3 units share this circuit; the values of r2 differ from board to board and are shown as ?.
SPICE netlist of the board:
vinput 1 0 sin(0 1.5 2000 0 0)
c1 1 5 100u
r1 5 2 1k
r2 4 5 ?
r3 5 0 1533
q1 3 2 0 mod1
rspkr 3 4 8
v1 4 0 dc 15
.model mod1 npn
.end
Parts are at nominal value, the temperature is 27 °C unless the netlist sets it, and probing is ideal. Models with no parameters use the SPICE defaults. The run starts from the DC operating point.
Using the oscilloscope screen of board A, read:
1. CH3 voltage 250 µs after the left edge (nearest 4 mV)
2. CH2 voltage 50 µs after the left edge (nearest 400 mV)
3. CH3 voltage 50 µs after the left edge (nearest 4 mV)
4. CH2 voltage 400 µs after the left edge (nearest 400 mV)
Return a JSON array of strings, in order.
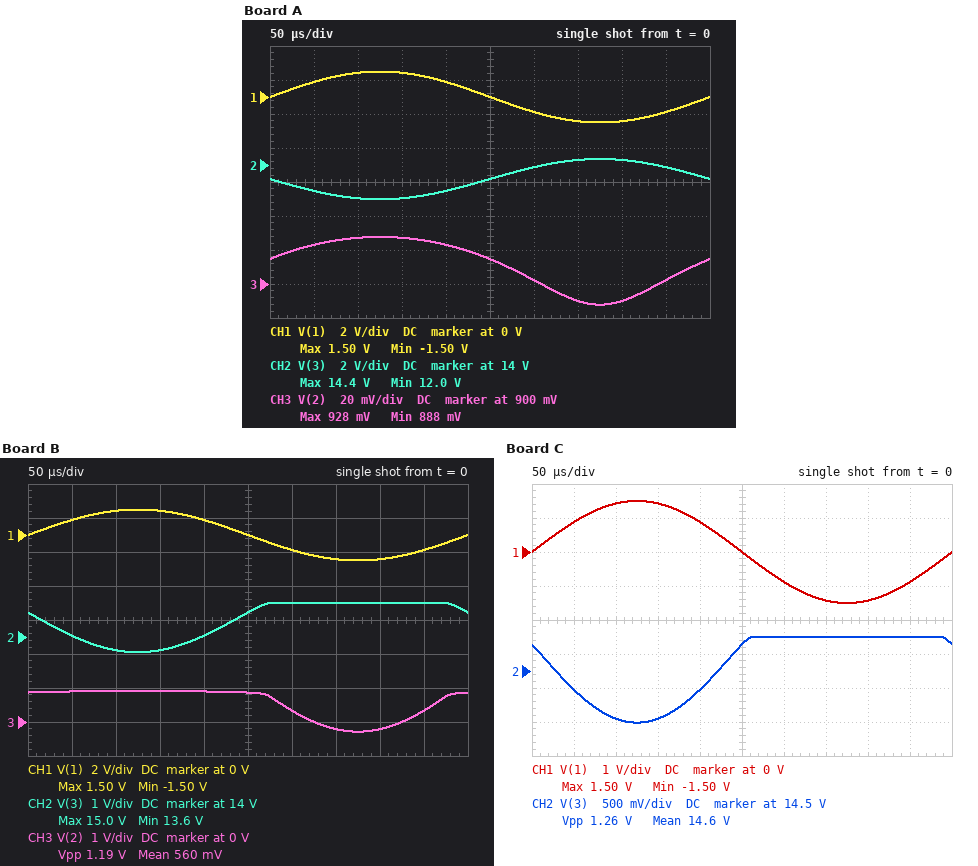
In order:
["916 mV", "12.4 V", "924 mV", "14.4 V"]
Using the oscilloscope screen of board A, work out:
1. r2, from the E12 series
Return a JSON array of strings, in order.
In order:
["2.7 kΩ"]
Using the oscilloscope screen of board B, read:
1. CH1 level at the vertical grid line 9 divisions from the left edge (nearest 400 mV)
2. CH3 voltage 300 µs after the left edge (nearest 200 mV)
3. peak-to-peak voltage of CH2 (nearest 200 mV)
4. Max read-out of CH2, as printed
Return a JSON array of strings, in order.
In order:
["-800 mV", "400 mV", "1.4 V", "15.0 V"]
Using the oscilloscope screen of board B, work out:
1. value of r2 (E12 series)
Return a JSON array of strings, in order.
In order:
["12 kΩ"]
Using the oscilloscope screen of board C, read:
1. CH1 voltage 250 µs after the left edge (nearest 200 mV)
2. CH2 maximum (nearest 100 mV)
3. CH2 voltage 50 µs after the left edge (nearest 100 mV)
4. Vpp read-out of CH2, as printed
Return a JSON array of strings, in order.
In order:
["0 V", "15.0 V", "14.2 V", "1.26 V"]
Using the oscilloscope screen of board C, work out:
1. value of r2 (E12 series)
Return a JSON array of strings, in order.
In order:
["18 kΩ"]
